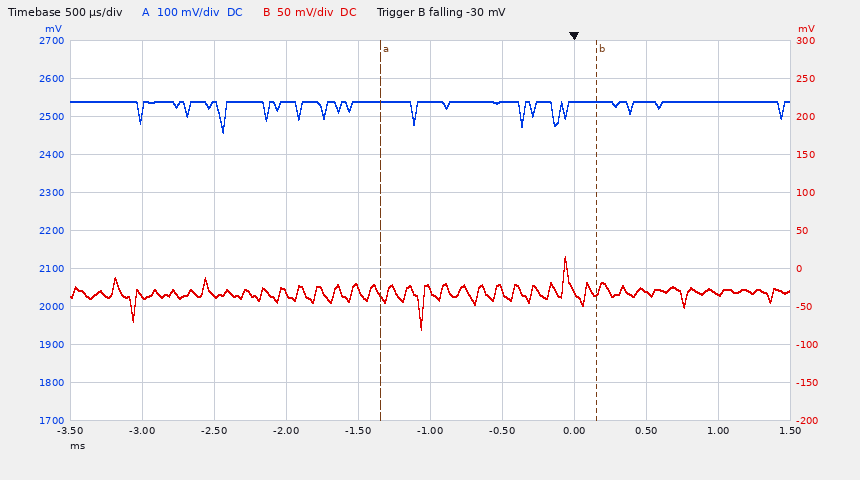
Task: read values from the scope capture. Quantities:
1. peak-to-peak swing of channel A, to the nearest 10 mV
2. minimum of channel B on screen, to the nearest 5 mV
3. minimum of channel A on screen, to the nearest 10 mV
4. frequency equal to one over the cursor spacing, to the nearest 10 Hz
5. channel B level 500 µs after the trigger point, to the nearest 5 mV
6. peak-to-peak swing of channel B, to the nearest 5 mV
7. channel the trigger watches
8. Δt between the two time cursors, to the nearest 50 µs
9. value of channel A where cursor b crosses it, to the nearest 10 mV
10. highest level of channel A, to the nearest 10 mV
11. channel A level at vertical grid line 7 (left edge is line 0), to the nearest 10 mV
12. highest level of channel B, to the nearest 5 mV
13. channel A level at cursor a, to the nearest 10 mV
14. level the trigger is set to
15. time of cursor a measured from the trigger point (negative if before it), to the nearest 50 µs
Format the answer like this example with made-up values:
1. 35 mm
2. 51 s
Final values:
1. 80 mV
2. -80 mV
3. 2.46 V
4. 670 Hz
5. -30 mV
6. 95 mV
7. channel B
8. 1.50 ms
9. 2.54 V
10. 2.54 V
11. 2.54 V
12. 15 mV
13. 2.54 V
14. -30 mV
15. -1.35 ms
